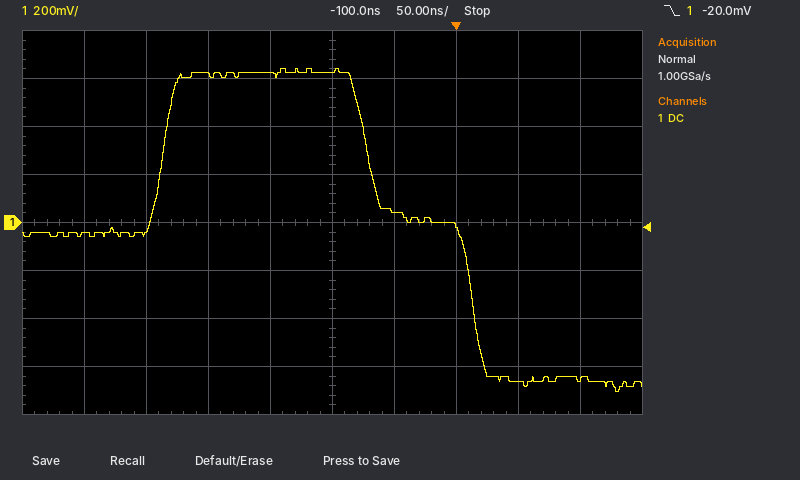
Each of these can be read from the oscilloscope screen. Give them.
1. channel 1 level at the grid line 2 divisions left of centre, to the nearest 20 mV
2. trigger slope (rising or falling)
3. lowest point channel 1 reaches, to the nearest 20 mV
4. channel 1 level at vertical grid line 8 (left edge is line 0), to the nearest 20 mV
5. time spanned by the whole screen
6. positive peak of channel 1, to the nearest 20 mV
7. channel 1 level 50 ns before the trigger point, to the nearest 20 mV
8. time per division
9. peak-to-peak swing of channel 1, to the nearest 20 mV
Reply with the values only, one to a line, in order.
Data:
620 mV
falling
-700 mV
-660 mV
500 ns
640 mV
40 mV
50 ns
1.34 V
